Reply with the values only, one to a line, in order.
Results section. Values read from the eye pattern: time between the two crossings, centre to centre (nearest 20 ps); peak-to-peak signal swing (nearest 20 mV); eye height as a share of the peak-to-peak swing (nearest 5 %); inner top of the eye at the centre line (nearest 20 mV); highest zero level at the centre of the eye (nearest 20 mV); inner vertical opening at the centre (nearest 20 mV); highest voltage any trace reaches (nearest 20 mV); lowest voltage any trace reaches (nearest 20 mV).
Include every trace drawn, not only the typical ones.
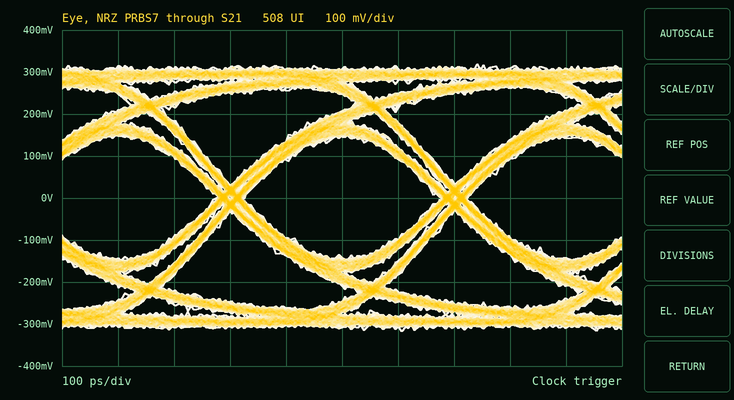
400 ps
640 mV
45 %
140 mV
-140 mV
280 mV
320 mV
-320 mV
